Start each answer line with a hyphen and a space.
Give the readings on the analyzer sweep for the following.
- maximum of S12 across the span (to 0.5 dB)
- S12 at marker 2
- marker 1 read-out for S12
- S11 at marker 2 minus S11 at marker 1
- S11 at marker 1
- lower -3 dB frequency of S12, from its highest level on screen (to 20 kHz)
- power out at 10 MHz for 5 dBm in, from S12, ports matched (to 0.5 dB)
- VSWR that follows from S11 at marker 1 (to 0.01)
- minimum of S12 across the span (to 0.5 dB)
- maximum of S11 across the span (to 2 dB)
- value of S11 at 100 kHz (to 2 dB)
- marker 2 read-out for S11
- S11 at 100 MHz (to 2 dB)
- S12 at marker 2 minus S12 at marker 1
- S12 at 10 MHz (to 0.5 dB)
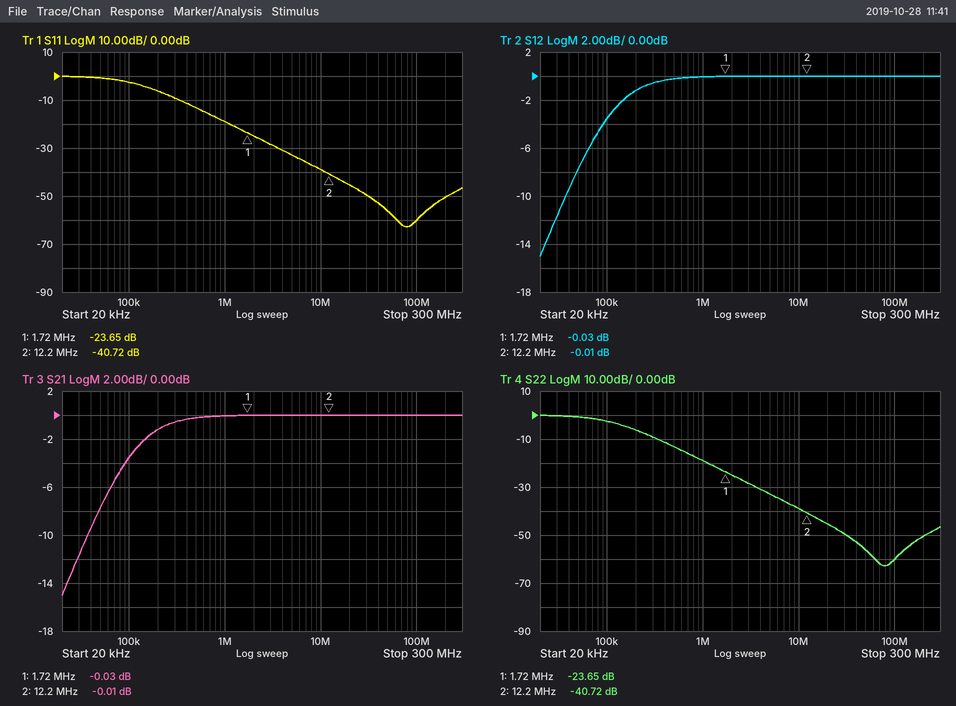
- 0.0 dB
- -0.01 dB
- -0.03 dB
- -17.07 dB
- -23.65 dB
- 120 kHz
- 5.0 dBm
- 1.14
- -15.0 dB
- 0 dB
- -2 dB
- -40.72 dB
- -60 dB
- 0.02 dB
- 0.0 dB
